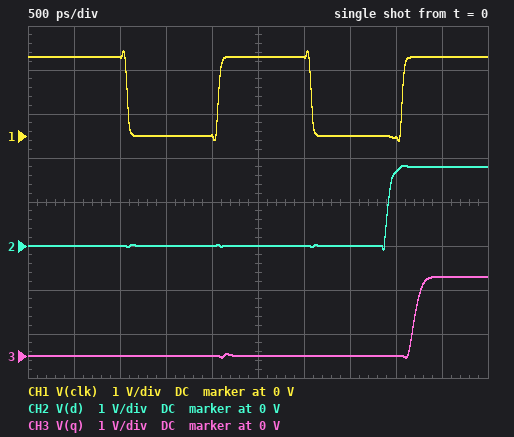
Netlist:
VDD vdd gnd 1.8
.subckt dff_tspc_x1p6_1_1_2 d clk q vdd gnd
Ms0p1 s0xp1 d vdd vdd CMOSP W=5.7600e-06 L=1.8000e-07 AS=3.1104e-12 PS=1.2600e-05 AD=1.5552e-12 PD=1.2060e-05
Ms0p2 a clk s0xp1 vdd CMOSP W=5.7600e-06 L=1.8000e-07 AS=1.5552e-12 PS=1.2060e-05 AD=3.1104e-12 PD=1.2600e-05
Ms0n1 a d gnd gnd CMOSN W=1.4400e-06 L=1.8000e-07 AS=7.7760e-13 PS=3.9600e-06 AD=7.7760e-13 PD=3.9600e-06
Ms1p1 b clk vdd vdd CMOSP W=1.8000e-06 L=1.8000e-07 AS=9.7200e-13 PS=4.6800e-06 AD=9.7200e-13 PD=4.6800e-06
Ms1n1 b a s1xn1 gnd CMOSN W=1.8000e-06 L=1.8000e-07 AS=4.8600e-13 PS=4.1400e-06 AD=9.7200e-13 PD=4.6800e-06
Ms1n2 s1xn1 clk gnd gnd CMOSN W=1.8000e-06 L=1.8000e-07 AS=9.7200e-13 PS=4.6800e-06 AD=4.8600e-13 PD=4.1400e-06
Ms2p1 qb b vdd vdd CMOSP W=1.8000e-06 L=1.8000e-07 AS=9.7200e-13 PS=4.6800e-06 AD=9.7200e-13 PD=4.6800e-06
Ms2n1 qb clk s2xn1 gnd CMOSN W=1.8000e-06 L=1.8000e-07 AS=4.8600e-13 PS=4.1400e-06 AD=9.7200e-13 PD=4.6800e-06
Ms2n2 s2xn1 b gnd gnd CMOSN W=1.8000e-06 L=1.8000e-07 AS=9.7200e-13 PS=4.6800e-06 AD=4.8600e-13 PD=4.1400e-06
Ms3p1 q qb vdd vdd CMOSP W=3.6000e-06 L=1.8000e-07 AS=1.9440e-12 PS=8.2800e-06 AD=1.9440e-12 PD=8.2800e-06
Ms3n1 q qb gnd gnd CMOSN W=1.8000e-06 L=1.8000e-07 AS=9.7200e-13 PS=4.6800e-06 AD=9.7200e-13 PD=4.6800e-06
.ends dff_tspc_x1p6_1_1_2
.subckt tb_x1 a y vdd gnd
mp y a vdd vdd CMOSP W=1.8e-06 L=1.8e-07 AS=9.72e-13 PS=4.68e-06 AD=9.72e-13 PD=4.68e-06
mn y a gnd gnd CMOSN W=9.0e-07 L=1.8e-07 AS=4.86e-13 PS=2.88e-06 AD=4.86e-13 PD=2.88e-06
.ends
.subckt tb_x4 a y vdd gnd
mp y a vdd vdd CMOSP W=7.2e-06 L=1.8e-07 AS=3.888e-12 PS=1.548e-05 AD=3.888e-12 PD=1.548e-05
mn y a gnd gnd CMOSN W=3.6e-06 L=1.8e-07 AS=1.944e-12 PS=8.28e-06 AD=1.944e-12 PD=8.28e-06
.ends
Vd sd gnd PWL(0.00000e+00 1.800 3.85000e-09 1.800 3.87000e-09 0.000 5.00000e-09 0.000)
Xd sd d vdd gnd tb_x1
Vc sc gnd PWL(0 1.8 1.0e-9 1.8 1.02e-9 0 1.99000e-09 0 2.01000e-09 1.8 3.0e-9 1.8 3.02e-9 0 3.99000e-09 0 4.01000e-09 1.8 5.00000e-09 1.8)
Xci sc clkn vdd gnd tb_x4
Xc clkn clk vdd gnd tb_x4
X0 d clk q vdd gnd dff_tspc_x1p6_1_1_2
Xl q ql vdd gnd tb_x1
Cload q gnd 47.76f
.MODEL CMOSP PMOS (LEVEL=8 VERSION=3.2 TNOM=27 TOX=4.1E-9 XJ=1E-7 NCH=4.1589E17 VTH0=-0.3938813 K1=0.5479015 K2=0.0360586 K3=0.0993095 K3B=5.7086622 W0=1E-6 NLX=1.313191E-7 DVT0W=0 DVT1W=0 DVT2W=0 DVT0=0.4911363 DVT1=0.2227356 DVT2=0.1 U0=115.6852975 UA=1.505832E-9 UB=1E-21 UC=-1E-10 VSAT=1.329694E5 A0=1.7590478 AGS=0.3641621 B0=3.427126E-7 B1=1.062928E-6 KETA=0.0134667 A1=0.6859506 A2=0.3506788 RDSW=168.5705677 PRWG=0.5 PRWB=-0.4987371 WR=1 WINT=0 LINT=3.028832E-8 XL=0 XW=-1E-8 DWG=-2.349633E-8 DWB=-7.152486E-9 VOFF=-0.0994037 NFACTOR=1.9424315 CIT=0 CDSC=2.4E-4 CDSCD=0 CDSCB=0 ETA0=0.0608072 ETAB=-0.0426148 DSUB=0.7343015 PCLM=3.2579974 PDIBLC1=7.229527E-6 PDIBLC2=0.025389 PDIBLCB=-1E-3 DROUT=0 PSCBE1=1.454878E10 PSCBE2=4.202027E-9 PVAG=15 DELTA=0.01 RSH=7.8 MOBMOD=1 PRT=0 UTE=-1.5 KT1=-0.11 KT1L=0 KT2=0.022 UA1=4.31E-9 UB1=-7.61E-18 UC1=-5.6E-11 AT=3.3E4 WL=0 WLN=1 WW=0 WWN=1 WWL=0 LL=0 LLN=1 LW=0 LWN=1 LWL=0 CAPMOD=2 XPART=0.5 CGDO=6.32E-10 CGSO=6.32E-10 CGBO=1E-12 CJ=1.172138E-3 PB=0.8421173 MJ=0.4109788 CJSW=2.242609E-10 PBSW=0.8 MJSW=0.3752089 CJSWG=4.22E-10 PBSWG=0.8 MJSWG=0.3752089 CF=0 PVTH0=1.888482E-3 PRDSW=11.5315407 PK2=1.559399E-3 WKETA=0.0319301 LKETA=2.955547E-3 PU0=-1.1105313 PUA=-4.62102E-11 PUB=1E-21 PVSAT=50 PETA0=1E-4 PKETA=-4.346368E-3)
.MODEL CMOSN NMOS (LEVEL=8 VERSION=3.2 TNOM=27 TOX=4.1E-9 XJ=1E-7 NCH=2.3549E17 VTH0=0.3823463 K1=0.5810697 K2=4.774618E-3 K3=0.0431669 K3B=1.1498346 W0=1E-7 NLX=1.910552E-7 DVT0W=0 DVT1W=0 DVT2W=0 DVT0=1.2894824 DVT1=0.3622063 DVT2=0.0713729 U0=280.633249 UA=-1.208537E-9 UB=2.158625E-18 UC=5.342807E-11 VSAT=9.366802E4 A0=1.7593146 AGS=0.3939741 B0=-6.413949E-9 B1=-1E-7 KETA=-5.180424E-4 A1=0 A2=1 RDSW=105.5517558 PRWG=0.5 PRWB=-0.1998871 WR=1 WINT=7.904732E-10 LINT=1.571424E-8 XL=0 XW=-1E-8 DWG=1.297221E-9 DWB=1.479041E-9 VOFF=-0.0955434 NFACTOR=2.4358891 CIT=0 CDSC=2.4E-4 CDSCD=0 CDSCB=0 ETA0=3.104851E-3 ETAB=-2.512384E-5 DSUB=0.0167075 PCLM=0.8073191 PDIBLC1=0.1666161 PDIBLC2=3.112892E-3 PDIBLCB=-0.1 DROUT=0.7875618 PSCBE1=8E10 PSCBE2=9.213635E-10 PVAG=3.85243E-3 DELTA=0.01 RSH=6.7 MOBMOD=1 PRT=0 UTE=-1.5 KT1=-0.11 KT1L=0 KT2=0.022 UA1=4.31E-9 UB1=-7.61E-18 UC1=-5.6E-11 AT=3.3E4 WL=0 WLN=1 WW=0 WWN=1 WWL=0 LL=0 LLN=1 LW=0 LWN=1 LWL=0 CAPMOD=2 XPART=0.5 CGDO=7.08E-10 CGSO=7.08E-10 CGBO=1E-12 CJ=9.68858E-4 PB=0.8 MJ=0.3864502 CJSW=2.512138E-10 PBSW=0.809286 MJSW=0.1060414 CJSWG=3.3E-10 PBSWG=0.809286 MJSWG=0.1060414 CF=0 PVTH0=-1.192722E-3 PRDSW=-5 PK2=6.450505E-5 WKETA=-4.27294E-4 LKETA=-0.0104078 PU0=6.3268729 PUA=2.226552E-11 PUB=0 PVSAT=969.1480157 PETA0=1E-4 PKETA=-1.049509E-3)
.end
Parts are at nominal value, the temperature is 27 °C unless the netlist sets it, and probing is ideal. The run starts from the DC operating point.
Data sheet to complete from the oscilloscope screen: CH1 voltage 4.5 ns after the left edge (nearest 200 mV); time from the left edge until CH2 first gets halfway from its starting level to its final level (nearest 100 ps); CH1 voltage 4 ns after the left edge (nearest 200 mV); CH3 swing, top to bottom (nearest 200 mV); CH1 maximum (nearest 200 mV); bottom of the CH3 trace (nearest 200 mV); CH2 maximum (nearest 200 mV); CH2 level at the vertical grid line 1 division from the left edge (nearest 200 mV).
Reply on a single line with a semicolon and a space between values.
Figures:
1.8 V; 3.9 ns; 0 V; 1.8 V; 2.0 V; 0 V; 1.8 V; 0 V
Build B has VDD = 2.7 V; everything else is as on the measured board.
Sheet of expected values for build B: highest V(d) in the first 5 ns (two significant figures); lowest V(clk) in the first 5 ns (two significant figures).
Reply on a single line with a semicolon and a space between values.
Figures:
2.7 V; -79 mV
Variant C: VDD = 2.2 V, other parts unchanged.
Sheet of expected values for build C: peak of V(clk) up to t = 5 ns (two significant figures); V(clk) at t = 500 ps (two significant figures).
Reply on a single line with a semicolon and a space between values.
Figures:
2.3 V; 2.2 V
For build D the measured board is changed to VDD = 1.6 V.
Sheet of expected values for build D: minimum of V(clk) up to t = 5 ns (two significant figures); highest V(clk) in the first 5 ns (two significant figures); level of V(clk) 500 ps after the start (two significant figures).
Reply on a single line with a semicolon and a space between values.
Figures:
-160 mV; 1.7 V; 1.6 V
